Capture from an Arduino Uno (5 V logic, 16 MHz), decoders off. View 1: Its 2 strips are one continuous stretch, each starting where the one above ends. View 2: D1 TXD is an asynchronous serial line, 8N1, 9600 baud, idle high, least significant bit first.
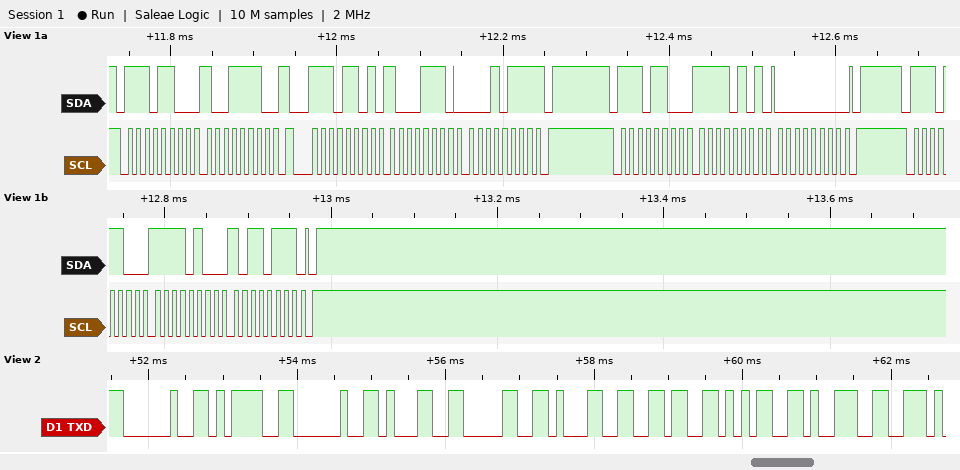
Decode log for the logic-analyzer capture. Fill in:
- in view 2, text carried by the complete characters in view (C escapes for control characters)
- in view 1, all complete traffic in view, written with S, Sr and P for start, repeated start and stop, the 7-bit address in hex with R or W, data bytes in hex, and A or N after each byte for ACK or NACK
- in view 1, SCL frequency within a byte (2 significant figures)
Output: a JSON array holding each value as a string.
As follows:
["\" = 101659\"", "S 76W A 9E A Sr 76R A 8E A 17 N P S 76W A F5 A 00 A P S 76W A F4 A B7 A P", "100 kHz"]
